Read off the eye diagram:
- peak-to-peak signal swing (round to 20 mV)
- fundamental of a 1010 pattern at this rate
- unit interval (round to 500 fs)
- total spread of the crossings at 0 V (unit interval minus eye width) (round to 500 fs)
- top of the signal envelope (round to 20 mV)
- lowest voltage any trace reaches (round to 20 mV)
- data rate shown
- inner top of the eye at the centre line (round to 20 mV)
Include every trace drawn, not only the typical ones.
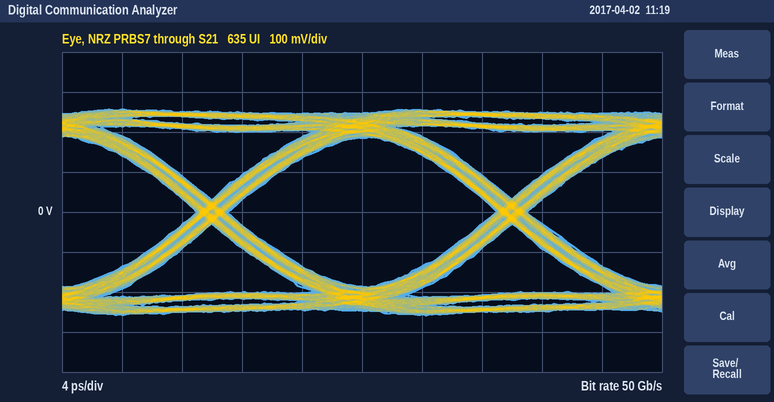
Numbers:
520 mV
25 GHz
20.0 ps
2.0 ps
260 mV
-260 mV
50 Gb/s
180 mV
